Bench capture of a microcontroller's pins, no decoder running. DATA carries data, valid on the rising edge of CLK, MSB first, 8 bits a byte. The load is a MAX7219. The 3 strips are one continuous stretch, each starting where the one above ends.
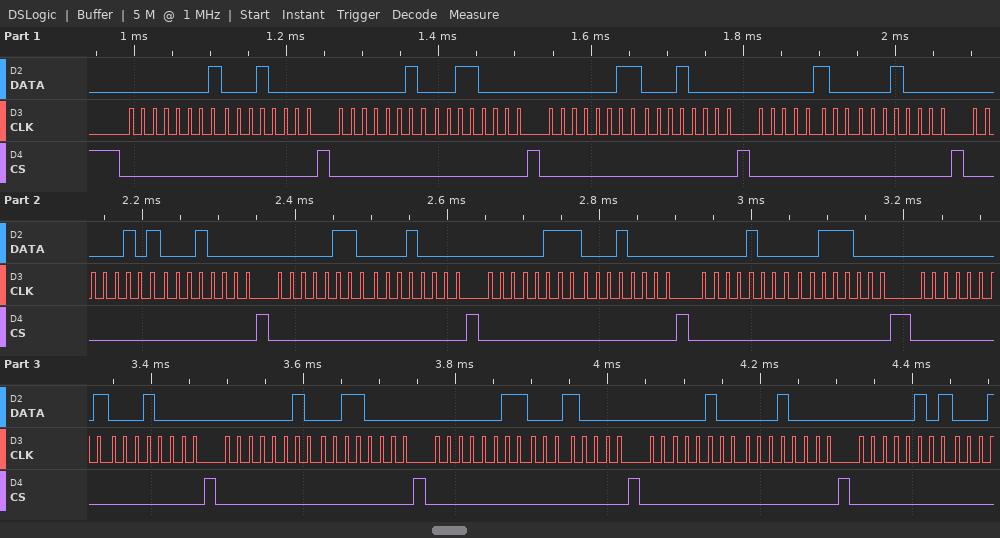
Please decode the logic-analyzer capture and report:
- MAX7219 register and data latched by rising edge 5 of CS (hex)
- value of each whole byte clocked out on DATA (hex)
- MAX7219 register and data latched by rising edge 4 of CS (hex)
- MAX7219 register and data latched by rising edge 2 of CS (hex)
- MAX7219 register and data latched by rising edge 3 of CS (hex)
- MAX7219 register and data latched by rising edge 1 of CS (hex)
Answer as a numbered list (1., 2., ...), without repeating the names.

1. register 0x5, data 0x10
2. 01 10 02 30 03 10 04 10 05 10 06 10 07 10 08 38 01 10 02 30 03 10 04 10 05
3. register 0x4, data 0x10
4. register 0x2, data 0x30
5. register 0x3, data 0x10
6. register 0x1, data 0x10
